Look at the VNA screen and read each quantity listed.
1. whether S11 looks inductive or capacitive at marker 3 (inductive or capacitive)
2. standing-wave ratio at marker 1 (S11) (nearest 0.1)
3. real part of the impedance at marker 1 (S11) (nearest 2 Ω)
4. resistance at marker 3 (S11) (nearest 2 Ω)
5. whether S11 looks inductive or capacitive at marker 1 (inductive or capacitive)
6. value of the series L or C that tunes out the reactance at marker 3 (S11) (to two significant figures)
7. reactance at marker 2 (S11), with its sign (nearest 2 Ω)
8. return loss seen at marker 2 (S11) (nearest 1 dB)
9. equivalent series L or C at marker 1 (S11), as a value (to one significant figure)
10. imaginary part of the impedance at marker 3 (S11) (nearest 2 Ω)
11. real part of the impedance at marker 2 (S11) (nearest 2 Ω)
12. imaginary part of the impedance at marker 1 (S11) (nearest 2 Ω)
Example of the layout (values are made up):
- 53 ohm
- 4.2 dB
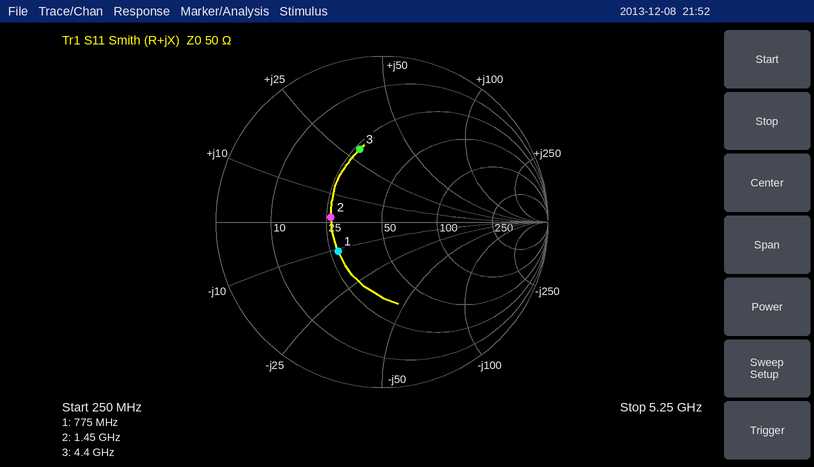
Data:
- inductive
- 1.9
- 28 Ω
- 26 Ω
- capacitive
- 1.2 pF
- +2 Ω
- 10 dB
- 20 pF
- +30 Ω
- 26 Ω
- -10 Ω
